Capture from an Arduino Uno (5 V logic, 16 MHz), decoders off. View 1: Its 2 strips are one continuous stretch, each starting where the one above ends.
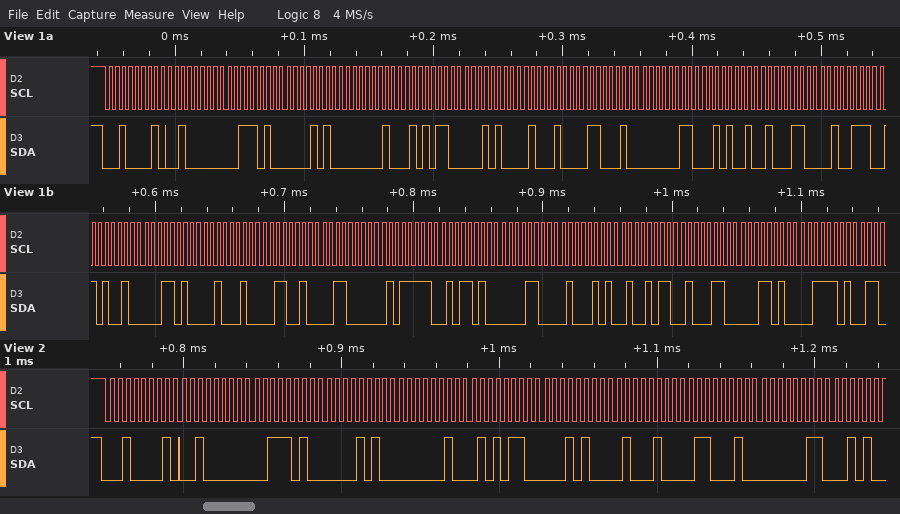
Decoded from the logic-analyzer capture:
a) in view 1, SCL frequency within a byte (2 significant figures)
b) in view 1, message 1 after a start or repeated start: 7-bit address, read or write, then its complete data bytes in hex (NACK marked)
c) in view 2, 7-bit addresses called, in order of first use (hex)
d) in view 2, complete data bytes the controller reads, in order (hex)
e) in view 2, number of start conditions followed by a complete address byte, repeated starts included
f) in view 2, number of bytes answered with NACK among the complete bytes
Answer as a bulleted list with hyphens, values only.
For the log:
- 200 kHz
- 0x10 read: 20 3A 0A 02 56 14 44 62 03 29 46 27 52 1A 22 32 30 5F 5A 0C 45 4B 46 1A 3D
- 0x10
- 20 3A 0A 02 56 14 44 62 03
- 1
- 0
